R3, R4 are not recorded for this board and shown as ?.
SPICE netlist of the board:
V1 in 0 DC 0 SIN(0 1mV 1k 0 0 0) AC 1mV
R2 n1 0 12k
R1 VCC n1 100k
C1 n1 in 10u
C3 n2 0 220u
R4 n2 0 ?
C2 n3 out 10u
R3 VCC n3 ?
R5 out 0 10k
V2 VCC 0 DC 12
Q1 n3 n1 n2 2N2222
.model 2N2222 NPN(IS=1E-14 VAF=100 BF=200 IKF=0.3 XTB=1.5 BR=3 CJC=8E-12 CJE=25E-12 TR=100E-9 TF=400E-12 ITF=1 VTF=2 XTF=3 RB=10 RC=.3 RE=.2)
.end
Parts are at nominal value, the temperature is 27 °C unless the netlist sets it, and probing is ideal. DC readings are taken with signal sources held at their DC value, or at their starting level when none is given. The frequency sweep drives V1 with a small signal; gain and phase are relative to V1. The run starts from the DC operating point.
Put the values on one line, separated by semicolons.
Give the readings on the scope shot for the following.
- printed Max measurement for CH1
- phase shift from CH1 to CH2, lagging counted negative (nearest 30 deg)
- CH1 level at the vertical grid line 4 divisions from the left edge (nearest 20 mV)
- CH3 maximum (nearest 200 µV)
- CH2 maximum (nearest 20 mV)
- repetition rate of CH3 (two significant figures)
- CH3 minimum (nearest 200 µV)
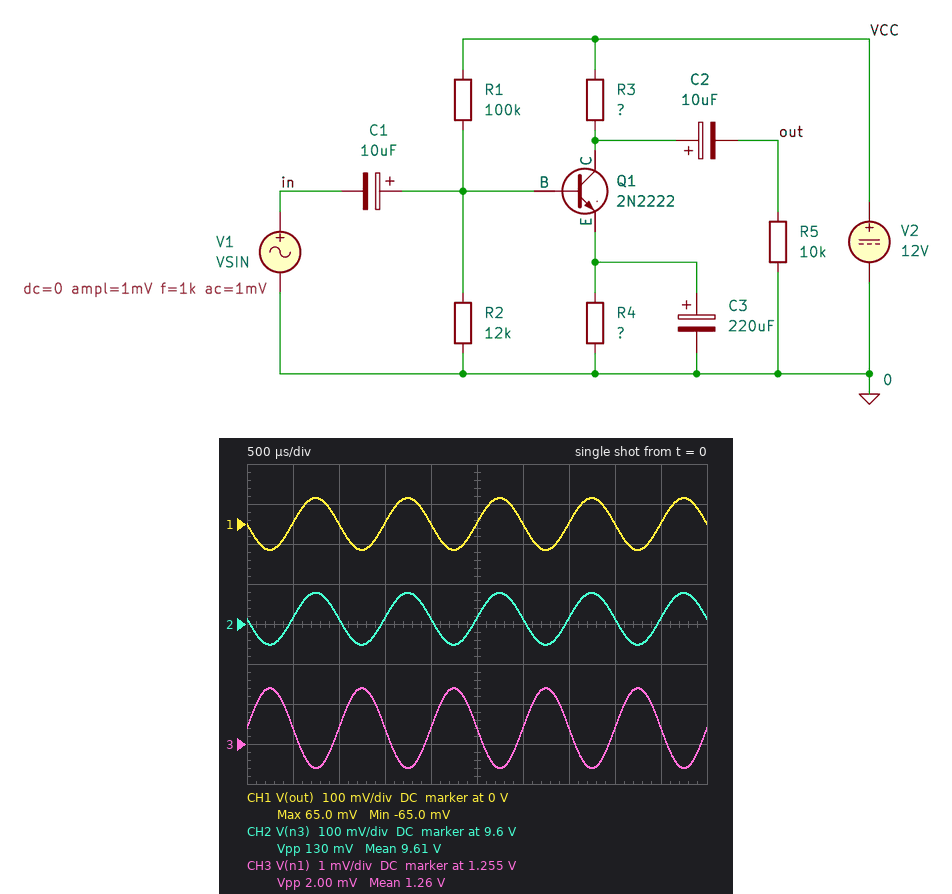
65.0 mV; 0 deg; 0 V; 1.2564 V; 9.68 V; 1.0 kHz; 1.2544 V
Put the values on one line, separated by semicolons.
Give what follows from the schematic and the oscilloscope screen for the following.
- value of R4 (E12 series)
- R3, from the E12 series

1 kΩ; 3.9 kΩ
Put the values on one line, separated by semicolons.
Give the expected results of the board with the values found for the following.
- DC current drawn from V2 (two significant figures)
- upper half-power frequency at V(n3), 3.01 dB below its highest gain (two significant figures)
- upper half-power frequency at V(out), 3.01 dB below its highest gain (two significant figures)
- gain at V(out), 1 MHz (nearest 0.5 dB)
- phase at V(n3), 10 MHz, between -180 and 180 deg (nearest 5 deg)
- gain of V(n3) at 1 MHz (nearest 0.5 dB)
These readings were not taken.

720 µA; 13 MHz; 13 MHz; 36.0 dB; 140 deg; 36.0 dB
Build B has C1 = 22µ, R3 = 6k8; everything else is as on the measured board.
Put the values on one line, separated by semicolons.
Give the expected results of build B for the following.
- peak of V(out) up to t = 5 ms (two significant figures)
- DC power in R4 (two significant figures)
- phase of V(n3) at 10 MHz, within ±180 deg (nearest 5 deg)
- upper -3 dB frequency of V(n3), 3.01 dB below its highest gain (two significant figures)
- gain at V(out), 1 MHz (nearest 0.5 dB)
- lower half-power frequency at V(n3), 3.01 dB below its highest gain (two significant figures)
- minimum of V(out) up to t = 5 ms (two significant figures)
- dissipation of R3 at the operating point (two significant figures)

93 mV; 380 µW; 130 deg; 8.6 MHz; 39.5 dB; 18 Hz; -93 mV; 2.5 mW
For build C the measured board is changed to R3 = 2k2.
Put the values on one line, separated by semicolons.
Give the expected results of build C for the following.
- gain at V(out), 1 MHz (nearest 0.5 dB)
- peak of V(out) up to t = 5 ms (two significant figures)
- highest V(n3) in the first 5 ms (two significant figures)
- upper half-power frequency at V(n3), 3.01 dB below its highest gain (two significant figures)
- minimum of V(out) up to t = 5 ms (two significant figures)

32.5 dB; 42 mV; 11 V; 21 MHz; -42 mV
